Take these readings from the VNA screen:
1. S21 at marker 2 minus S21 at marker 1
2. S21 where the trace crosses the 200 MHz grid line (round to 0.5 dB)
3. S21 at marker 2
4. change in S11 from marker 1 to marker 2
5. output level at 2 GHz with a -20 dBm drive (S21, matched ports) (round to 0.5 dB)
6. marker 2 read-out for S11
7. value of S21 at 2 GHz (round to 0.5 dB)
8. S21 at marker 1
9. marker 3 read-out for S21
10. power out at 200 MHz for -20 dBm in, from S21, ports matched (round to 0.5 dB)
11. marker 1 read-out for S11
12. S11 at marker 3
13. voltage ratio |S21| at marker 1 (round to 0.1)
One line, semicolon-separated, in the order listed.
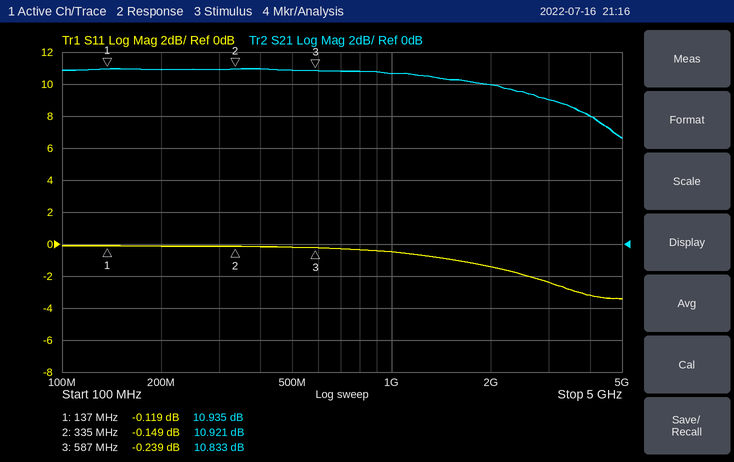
-0.014 dB; 11.0 dB; 10.921 dB; -0.030 dB; -10.0 dBm; -0.149 dB; 10.0 dB; 10.935 dB; 10.833 dB; -9.0 dBm; -0.119 dB; -0.239 dB; 3.5
